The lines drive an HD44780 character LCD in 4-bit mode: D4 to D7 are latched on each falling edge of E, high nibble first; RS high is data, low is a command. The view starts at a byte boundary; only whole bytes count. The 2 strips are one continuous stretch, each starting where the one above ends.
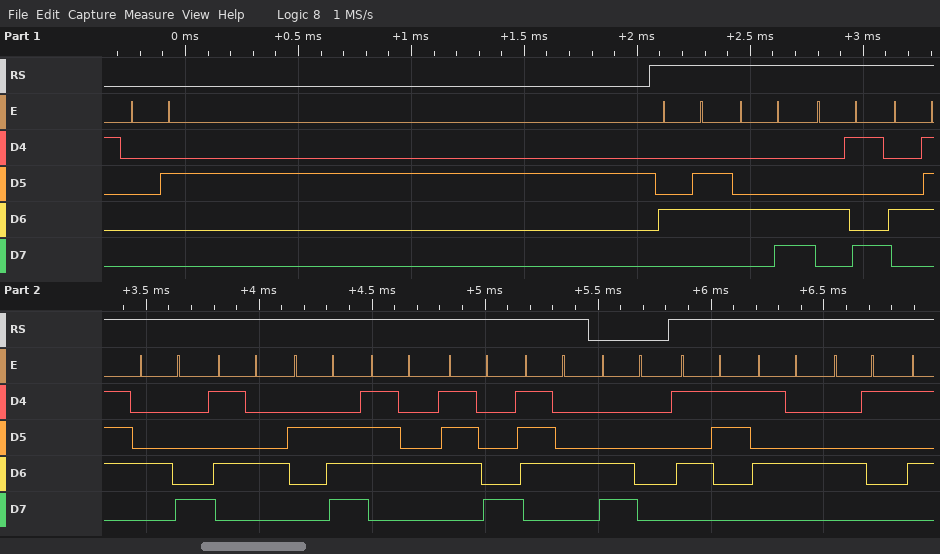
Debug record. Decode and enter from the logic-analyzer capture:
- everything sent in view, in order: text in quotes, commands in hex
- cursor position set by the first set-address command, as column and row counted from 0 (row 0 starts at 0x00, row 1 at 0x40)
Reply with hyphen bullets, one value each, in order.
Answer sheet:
- 0x02 "FLIGHT.txt" 0xC0 "STA"
- column 0, row 1
